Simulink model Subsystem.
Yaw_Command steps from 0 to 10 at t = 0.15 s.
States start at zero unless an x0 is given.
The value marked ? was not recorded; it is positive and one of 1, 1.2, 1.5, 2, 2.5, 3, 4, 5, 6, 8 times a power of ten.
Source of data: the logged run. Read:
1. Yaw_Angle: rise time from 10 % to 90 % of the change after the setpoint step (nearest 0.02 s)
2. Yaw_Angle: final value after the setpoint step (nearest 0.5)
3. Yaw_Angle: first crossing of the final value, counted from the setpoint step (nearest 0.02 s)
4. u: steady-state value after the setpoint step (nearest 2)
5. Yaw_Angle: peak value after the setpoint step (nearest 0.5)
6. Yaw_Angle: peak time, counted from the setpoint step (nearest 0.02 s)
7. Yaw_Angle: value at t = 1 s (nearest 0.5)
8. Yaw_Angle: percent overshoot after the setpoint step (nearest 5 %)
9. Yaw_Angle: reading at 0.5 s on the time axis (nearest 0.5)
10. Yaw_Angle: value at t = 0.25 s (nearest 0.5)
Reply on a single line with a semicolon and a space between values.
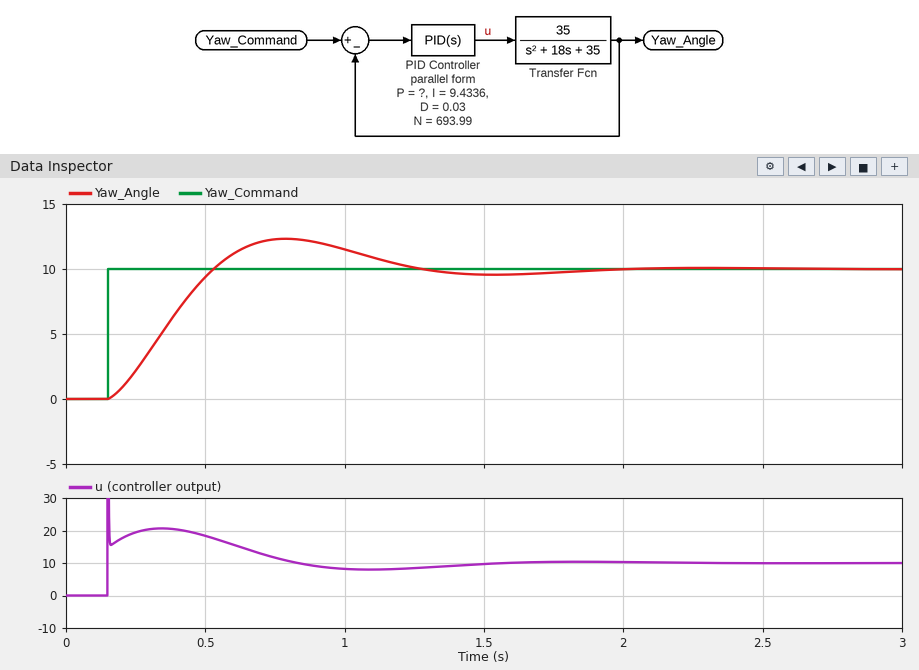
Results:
0.28 s; 10.0; 0.38 s; 10; 12.5; 0.64 s; 11.5; 25 %; 9.5; 2.0
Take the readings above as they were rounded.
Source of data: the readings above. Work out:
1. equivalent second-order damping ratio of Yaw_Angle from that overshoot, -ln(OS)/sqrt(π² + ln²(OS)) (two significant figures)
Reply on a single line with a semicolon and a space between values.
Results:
0.40
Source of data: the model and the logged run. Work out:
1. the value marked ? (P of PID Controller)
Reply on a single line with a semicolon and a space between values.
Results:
1.5
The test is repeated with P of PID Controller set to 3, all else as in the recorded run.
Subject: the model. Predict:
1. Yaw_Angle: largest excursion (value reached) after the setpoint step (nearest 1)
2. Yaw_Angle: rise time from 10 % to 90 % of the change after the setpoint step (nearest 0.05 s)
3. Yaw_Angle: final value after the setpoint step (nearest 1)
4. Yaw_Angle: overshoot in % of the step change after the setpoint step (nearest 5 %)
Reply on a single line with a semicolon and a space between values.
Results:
11; 0.20 s; 10; 10 %
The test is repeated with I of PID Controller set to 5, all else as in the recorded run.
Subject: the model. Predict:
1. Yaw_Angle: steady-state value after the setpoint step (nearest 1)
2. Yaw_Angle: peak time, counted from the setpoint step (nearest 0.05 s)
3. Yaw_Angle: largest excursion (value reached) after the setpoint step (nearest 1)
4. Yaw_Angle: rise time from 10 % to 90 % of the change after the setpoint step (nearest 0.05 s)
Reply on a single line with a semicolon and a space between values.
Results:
10; 0.90 s; 11; 0.40 s
